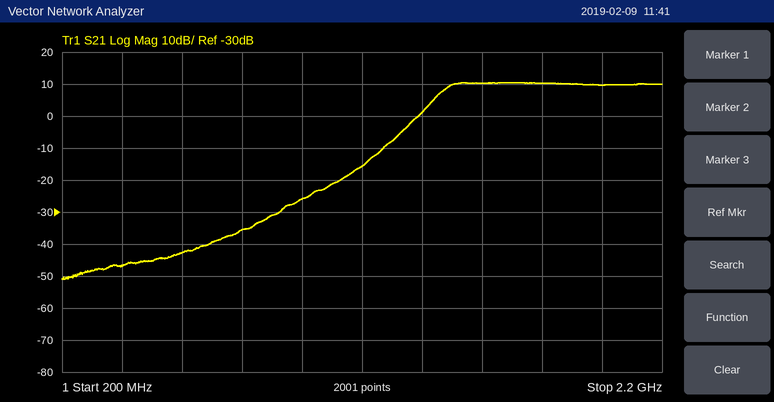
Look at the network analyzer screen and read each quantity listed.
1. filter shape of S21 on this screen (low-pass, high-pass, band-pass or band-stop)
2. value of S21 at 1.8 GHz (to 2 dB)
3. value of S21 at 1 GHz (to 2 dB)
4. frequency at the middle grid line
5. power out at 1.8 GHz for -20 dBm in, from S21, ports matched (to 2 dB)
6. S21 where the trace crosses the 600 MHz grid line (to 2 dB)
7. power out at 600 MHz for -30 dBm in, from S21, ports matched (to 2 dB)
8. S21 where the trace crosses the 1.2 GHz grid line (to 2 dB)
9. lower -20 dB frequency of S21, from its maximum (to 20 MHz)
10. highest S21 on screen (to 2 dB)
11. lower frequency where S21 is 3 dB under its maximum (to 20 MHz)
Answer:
high-pass
10 dB
-26 dB
1.2 GHz
-10 dBm
-42 dB
-72 dBm
-16 dB
1.28 GHz
10 dB
1.46 GHz
